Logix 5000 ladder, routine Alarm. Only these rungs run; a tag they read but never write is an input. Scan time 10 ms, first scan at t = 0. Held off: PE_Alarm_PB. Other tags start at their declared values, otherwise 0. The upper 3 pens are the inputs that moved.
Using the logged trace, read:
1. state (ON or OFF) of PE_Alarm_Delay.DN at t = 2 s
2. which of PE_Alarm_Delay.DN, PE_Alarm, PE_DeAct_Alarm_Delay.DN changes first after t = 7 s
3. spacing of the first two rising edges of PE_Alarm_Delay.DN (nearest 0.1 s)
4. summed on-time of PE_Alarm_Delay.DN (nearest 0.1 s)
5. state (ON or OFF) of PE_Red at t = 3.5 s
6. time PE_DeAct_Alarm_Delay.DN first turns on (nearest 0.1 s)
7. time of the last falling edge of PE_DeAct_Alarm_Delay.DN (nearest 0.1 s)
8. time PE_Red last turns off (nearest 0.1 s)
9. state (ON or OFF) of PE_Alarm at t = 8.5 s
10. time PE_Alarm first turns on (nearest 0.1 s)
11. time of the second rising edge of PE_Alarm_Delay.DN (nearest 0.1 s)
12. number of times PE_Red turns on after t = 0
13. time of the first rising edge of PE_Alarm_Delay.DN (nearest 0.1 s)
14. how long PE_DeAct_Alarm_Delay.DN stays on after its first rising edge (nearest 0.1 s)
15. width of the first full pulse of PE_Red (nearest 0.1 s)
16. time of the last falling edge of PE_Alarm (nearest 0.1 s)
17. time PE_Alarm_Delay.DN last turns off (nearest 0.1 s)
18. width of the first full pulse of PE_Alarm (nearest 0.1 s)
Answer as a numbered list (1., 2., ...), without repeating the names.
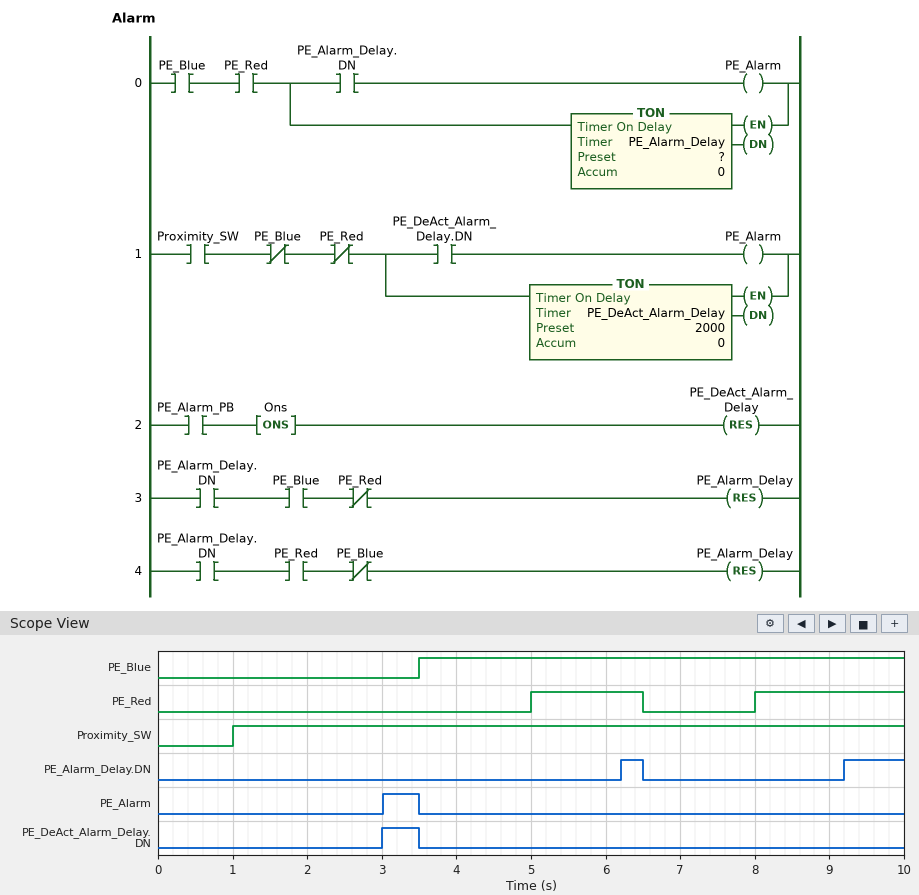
1. OFF
2. PE_Alarm_Delay.DN
3. 3.0 s
4. 1.1 s
5. OFF
6. 3.0 s
7. 3.5 s
8. 6.5 s
9. OFF
10. 3.0 s
11. 9.2 s
12. 2
13. 6.2 s
14. 0.5 s
15. 1.5 s
16. 3.5 s
17. 6.5 s
18. 0.5 s
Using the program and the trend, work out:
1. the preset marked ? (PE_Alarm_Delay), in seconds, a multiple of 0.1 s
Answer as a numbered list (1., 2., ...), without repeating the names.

1. 1.2 s
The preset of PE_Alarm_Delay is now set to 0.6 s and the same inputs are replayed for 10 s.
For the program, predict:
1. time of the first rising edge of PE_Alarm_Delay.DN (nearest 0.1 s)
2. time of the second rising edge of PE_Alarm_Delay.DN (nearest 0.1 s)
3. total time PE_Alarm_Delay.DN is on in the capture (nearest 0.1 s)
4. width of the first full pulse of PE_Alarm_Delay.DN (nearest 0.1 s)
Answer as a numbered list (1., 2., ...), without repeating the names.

1. 5.6 s
2. 8.6 s
3. 2.3 s
4. 0.9 s
